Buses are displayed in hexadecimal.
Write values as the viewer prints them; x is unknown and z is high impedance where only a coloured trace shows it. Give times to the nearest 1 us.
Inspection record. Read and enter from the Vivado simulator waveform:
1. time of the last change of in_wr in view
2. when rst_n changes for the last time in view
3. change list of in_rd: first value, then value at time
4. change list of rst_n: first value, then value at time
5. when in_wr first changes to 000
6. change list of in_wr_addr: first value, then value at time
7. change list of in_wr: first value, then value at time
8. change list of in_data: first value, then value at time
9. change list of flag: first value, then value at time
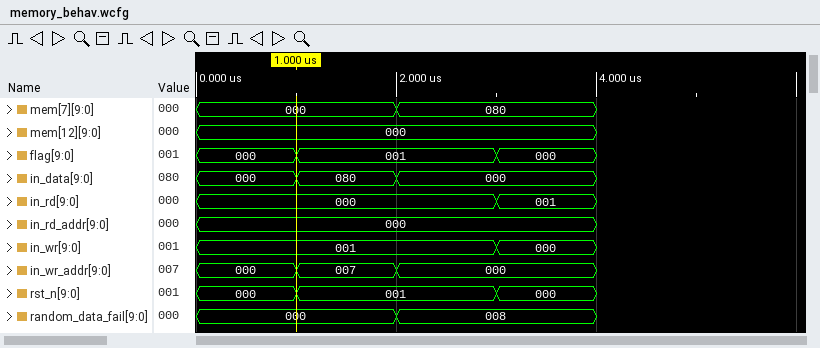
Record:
3 us
3 us
000, 001 at 3 us
000, 001 at 1 us, 000 at 3 us
3 us
000, 007 at 1 us, 000 at 2 us
001, 000 at 3 us
000, 080 at 1 us, 000 at 2 us
000, 001 at 1 us, 000 at 3 us
